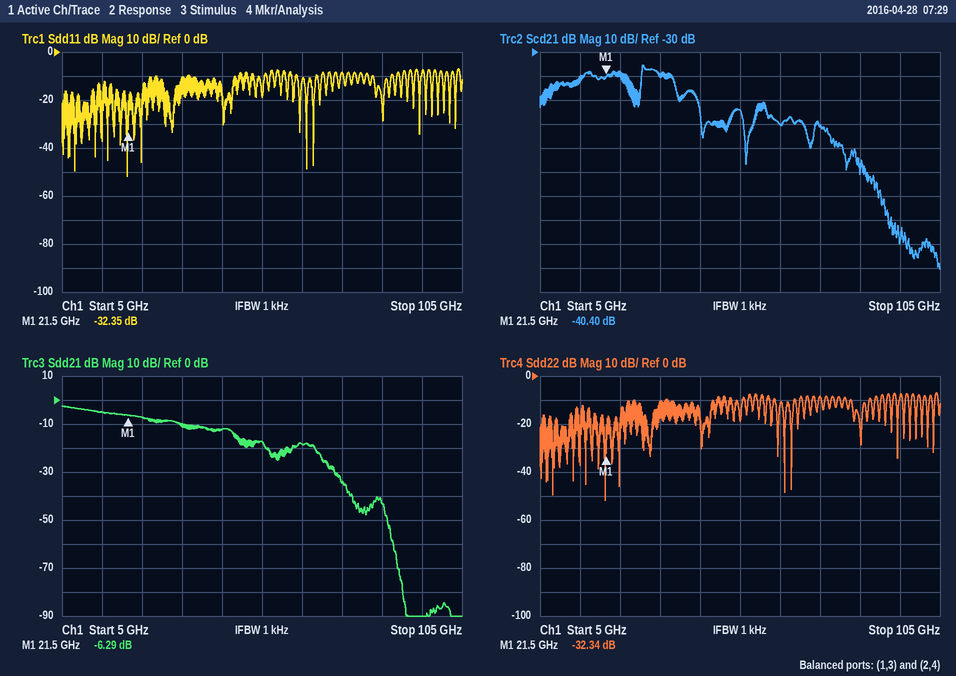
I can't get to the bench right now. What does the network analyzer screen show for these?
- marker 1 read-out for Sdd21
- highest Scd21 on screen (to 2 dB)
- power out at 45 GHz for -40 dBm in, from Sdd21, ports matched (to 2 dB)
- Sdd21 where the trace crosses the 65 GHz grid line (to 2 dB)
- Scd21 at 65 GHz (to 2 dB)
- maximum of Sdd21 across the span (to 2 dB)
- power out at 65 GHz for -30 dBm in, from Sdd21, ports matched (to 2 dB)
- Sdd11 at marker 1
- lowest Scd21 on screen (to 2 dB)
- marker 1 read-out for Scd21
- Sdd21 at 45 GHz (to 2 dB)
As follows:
-6.29 dB
-36 dB
-52 dBm
-18 dB
-60 dB
-2 dB
-48 dBm
-32.35 dB
-120 dB
-40.40 dB
-12 dB
